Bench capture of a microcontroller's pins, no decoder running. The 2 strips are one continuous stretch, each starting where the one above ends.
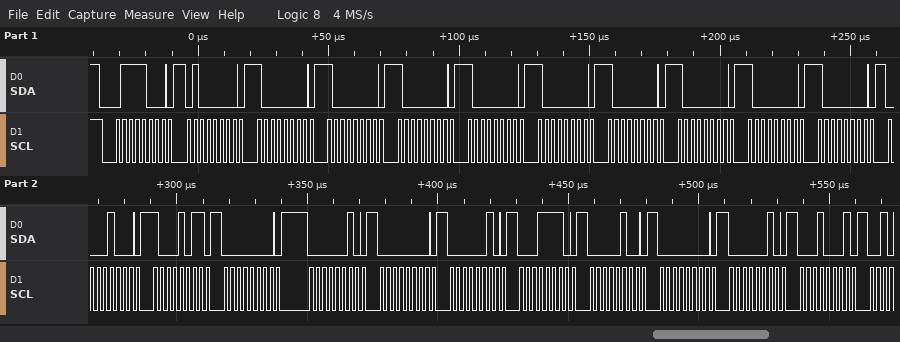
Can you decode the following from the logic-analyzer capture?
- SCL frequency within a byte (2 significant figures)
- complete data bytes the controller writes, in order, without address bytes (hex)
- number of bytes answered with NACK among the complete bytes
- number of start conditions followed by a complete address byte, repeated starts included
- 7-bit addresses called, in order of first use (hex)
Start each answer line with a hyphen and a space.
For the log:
- 400 kHz
- 40 80 80 80 80 80 80 80 80 80 08 8B 00 02 00 02 1E 04 00 02 11
- 0
- 1
- 0x3C
